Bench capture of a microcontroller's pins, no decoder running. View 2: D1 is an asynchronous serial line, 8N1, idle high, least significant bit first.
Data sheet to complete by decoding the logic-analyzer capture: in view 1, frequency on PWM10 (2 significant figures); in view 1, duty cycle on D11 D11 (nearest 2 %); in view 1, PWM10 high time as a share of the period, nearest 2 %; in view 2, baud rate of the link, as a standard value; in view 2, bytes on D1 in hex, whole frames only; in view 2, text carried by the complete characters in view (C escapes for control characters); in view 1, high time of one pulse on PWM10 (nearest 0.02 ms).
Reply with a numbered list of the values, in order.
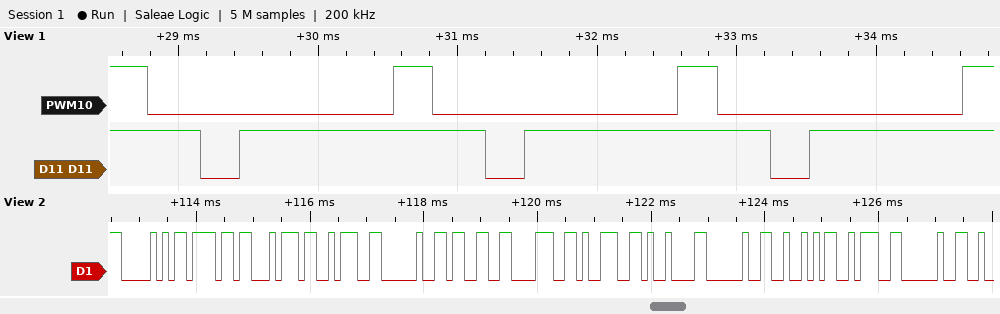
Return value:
1. 490 Hz
2. 86 %
3. 14 %
4. 9600 baud
5. 0x50 0x6F 0x74 0x3A 0x20 0x33 0x38 0x39 0x09 0x20 0x52 0x3A 0x20
6. "Pot: 389\t R: "
7. 0.28 ms
